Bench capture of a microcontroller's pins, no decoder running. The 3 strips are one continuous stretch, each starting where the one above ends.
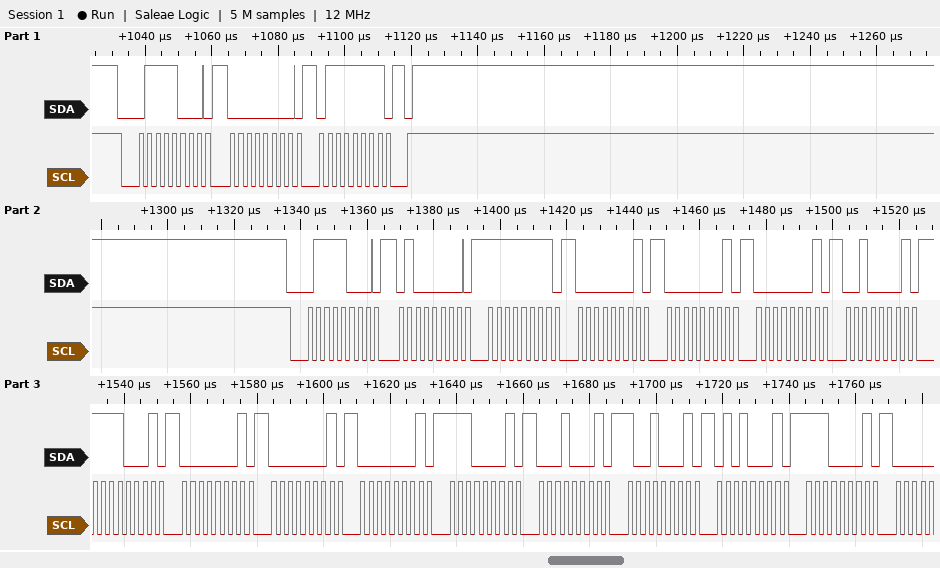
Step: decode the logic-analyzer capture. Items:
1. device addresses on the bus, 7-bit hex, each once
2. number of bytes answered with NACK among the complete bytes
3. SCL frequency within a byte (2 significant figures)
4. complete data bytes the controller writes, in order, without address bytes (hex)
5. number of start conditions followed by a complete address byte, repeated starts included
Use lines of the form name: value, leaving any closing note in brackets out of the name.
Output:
device addresses on the bus, 7-bit hex, each once: 0x3C
number of bytes answered with NACK among the complete bytes: 0
SCL frequency within a byte: 400 kHz
complete data bytes the controller writes, in order, without address bytes: 00 7F 40 FF 01 01 01 21 F1 01 01 01 E1 11 91 51 E1
number of start conditions followed by a complete address byte, repeated starts included: 2
